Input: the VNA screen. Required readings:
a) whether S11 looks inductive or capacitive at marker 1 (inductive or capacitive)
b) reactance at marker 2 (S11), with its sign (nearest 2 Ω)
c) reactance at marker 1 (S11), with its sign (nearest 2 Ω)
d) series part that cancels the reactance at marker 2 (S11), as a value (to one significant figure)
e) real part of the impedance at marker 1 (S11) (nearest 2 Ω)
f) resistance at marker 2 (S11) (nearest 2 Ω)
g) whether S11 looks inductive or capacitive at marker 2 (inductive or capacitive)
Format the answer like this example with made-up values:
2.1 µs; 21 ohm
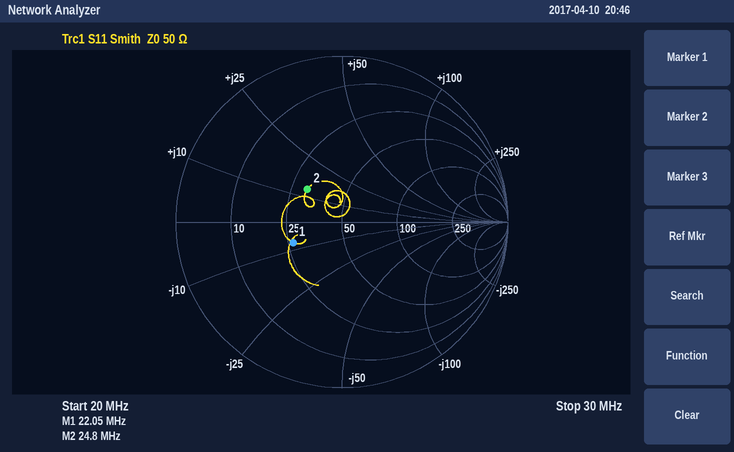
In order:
capacitive; +14 Ω; -8 Ω; 500 pF; 26 Ω; 30 Ω; inductive
